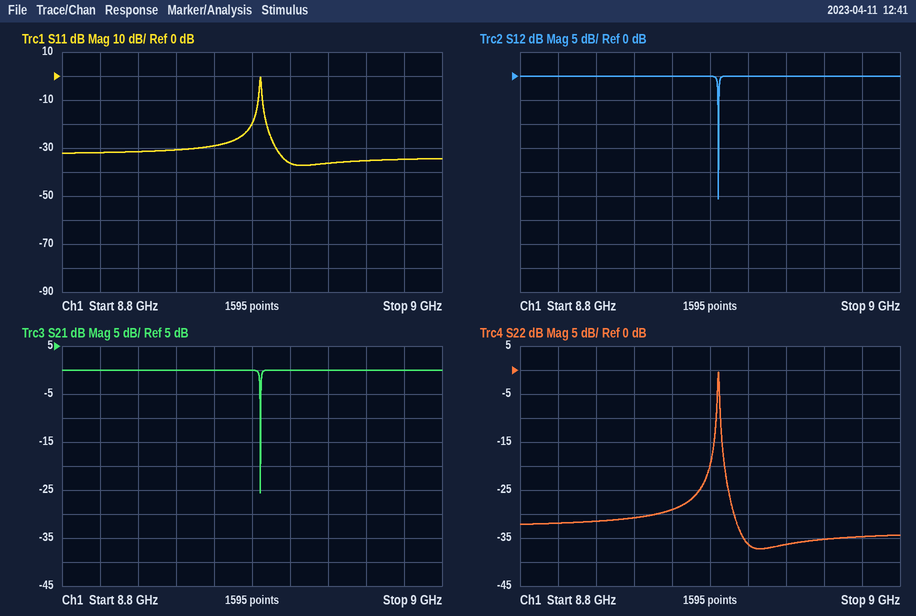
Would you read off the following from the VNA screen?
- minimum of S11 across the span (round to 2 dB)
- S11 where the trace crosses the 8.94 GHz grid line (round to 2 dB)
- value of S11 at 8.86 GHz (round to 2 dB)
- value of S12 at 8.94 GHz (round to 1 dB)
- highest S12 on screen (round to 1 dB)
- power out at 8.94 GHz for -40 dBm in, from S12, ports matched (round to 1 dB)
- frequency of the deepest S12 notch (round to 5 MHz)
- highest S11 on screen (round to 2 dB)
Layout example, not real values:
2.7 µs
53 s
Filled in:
-38 dB
-36 dB
-30 dB
0 dB
0 dB
-40 dBm
8.905 GHz
0 dB
